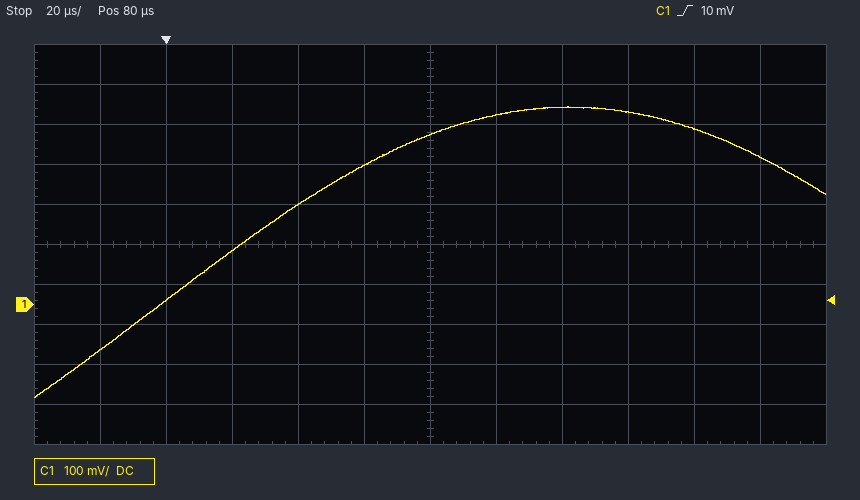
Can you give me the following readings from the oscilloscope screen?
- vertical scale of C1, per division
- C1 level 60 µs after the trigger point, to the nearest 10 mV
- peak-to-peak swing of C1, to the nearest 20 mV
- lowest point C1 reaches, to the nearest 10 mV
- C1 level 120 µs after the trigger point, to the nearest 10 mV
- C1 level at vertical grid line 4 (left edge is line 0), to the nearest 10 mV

100 mV
350 mV
720 mV
-230 mV
490 mV
250 mV
